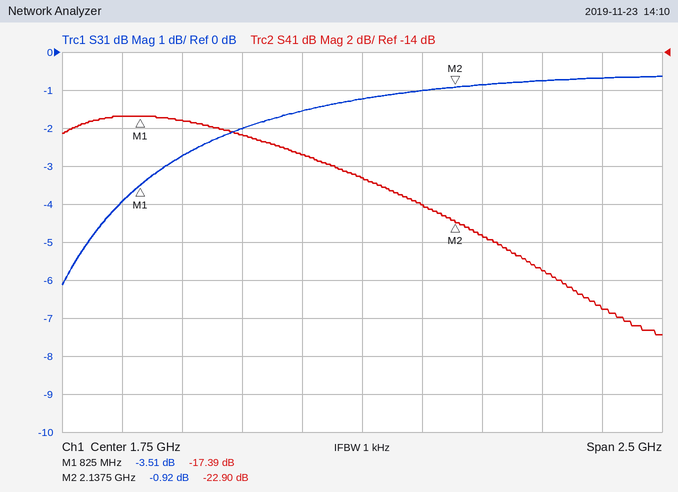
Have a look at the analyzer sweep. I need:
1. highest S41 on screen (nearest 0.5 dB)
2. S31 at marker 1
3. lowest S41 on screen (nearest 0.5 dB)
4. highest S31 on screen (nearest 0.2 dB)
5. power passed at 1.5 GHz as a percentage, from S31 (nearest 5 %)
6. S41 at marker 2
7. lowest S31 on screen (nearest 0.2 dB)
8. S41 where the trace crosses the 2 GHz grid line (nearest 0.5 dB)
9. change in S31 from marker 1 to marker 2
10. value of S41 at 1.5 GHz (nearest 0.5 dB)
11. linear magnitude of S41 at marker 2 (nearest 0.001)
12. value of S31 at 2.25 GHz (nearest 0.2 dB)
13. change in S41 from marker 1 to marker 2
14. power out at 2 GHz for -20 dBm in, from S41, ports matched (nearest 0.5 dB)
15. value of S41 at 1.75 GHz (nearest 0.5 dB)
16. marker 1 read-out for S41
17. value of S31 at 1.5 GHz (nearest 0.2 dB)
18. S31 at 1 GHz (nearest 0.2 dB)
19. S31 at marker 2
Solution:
-17.5 dB
-3.51 dB
-29.0 dB
-0.6 dB
70 %
-22.90 dB
-6.2 dB
-22.0 dB
2.59 dB
-19.5 dB
0.072
-0.8 dB
-5.51 dB
-42.0 dBm
-20.5 dB
-17.39 dB
-1.6 dB
-2.8 dB
-0.92 dB
